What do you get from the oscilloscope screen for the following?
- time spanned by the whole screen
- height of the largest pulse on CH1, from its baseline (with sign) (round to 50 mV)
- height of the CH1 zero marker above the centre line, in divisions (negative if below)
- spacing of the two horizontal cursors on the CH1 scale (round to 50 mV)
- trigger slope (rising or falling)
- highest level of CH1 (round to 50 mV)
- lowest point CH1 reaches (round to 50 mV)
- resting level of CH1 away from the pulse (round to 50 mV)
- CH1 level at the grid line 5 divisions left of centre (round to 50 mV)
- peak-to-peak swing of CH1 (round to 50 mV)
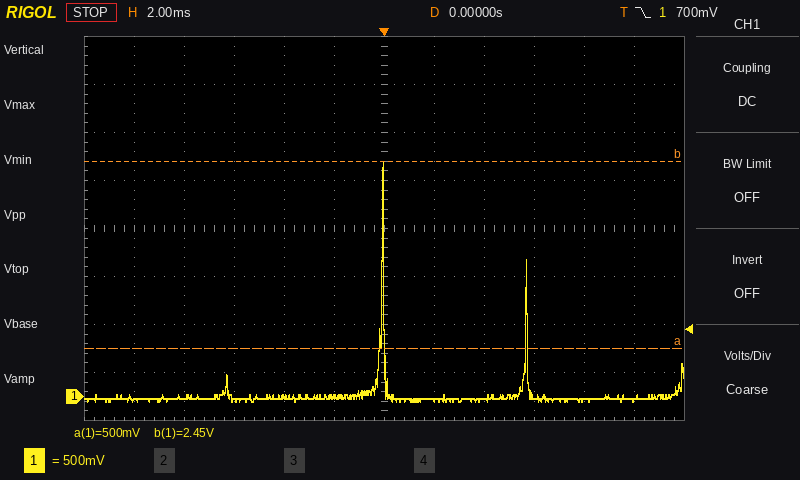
24 ms
+2.45 V
-3.5 div
1.95 V
falling
2.45 V
-50 mV
0 mV
-50 mV
2.50 V
